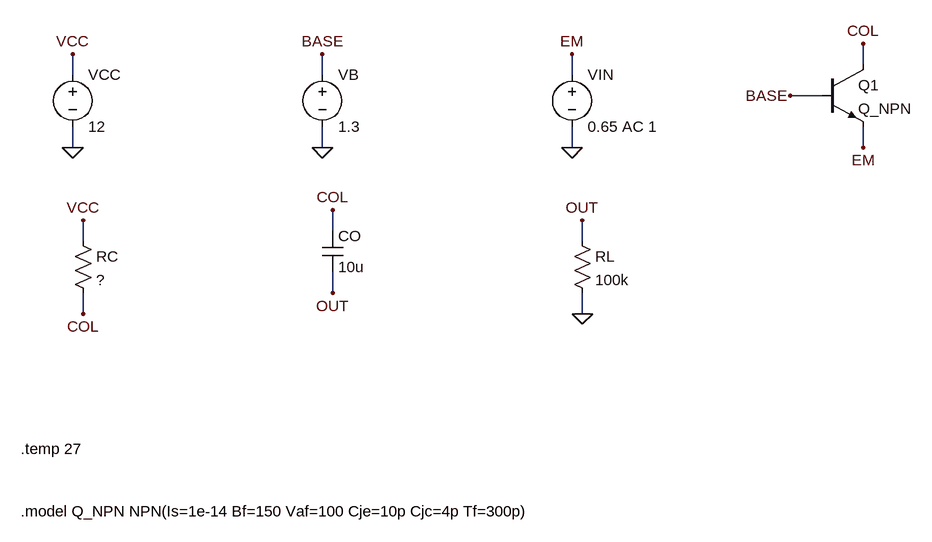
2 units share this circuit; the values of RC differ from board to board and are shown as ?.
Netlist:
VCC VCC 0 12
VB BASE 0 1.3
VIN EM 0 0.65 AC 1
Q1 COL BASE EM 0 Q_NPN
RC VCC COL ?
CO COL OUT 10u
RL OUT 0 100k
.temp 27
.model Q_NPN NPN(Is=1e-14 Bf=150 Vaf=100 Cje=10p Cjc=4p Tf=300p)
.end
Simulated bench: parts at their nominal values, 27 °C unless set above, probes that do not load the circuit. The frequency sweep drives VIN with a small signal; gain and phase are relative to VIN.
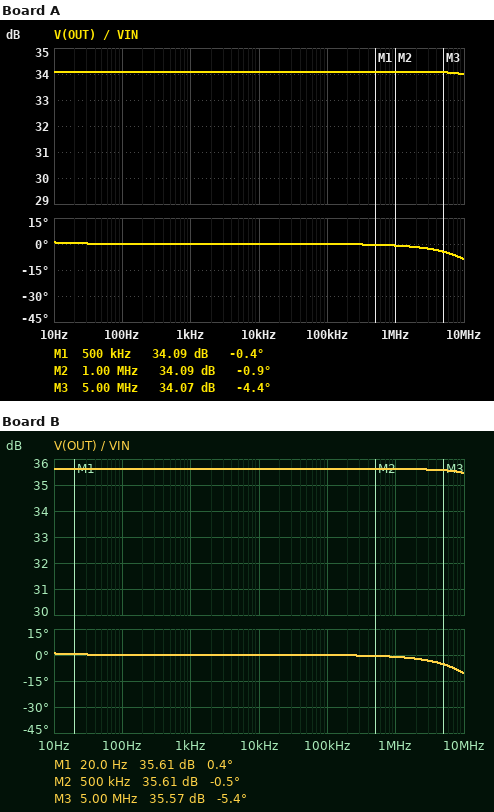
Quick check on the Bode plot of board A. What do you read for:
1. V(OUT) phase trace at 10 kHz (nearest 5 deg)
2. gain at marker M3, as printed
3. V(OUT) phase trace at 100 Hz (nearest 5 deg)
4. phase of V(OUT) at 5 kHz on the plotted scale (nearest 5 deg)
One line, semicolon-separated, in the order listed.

0 deg; 34.07 dB; 0 deg; 0 deg
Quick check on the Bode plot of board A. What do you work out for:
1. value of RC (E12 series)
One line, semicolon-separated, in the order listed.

1.5 kΩ
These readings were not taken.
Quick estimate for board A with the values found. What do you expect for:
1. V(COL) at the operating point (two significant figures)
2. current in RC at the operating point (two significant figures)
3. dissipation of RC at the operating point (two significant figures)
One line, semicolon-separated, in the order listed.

11 V; 900 µA; 1.2 mW
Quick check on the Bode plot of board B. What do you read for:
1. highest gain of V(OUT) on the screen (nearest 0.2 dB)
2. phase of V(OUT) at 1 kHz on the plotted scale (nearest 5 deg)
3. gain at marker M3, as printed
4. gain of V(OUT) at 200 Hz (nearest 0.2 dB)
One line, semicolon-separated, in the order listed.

35.6 dB; 0 deg; 35.57 dB; 35.6 dB
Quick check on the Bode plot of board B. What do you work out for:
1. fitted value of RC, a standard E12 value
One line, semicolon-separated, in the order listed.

1.8 kΩ
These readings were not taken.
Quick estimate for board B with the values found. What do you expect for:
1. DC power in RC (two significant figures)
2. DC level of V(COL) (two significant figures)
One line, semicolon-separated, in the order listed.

1.4 mW; 10 V
